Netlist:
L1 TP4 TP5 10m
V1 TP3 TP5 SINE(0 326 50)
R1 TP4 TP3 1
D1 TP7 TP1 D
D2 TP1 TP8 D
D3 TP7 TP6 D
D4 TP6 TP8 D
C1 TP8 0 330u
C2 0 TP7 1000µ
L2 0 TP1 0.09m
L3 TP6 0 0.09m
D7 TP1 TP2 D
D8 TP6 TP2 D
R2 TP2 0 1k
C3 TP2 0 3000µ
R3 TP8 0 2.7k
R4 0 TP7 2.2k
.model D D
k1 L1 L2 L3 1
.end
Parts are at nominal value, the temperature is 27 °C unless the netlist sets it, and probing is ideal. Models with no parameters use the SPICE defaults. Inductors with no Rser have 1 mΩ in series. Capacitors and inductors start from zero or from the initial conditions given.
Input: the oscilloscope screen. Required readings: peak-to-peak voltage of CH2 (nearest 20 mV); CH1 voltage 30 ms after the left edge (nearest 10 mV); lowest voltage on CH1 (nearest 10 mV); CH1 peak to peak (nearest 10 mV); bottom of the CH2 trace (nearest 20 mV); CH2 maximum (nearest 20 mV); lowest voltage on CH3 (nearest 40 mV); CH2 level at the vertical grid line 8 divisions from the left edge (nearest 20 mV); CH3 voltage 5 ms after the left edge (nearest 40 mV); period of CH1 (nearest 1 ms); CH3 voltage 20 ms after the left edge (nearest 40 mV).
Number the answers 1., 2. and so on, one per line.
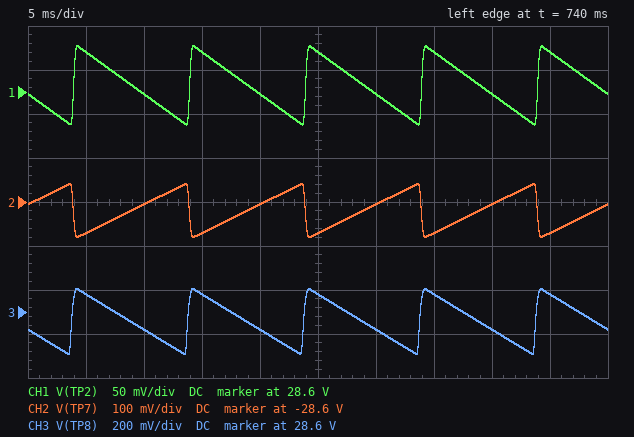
1. 120 mV
2. 28.60 V
3. 28.56 V
4. 90 mV
5. -28.68 V
6. -28.56 V
7. 28.40 V
8. -28.60 V
9. 28.68 V
10. 10 ms
11. 28.52 V
